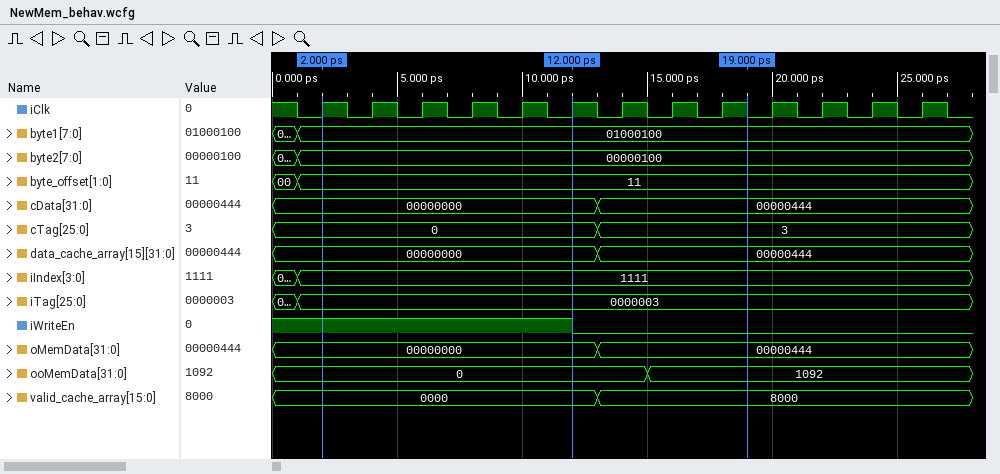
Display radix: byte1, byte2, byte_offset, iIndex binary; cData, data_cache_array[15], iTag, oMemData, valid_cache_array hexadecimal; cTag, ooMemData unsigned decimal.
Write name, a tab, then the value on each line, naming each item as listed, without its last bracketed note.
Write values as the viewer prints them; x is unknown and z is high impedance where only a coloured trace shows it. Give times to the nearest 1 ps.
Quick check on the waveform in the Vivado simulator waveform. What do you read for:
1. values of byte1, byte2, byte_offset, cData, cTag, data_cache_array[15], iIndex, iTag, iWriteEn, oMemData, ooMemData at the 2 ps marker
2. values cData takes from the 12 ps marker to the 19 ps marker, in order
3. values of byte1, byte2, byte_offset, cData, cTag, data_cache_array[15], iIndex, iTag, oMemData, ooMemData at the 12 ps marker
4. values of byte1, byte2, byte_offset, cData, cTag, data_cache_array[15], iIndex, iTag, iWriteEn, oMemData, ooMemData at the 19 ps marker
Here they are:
values of byte1, byte2, byte_offset, cData, cTag, data_cache_array[15], iIndex, iTag, iWriteEn, oMemData, ooMemData at the 2 ps marker	byte1=01000100, byte2=00000100, byte_offset=11, cData=00000000, cTag=0, data_cache_array[15]=00000000, iIndex=1111, iTag=0000003, iWriteEn=1, oMemData=00000000, ooMemData=0
values cData takes from the 12 ps marker to the 19 ps marker, in order	00000000, 00000444
values of byte1, byte2, byte_offset, cData, cTag, data_cache_array[15], iIndex, iTag, oMemData, ooMemData at the 12 ps marker	byte1=01000100, byte2=00000100, byte_offset=11, cData=00000000, cTag=0, data_cache_array[15]=00000000, iIndex=1111, iTag=0000003, oMemData=00000000, ooMemData=0
values of byte1, byte2, byte_offset, cData, cTag, data_cache_array[15], iIndex, iTag, iWriteEn, oMemData, ooMemData at the 19 ps marker	byte1=01000100, byte2=00000100, byte_offset=11, cData=00000444, cTag=3, data_cache_array[15]=00000444, iIndex=1111, iTag=0000003, iWriteEn=0, oMemData=00000444, ooMemData=1092
